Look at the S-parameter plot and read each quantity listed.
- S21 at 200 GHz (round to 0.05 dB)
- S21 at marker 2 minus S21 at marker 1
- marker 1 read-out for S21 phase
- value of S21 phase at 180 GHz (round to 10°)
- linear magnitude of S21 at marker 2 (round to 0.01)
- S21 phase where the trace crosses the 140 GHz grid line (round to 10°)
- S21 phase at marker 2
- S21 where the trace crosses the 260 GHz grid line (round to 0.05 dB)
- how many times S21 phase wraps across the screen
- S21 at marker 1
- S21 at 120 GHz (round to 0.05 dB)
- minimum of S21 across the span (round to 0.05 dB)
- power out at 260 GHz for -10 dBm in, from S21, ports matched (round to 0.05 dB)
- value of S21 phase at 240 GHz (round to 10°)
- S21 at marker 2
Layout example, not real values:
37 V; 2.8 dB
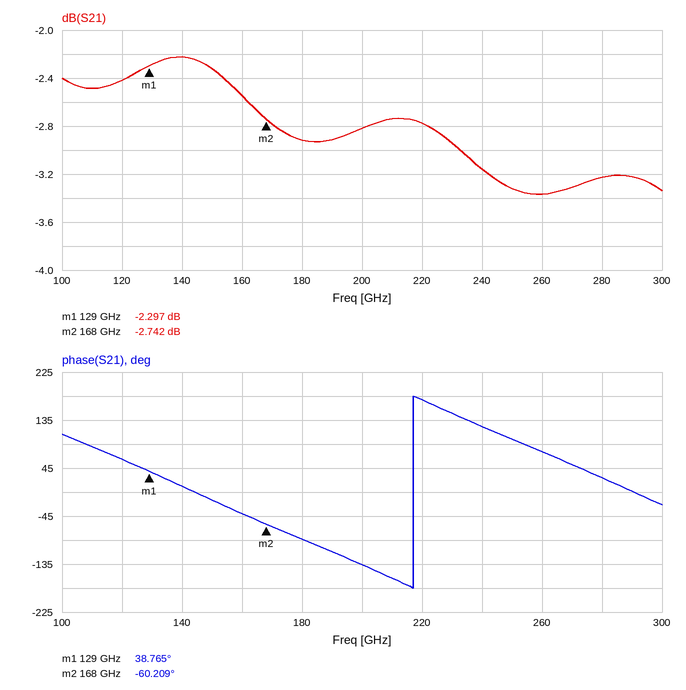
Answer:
-2.80 dB; -0.445 dB; 38.765°; -90°; 0.73; 10°; -60.209°; -3.35 dB; 1; -2.297 dB; -2.40 dB; -3.35 dB; -13.35 dBm; 120°; -2.742 dB
